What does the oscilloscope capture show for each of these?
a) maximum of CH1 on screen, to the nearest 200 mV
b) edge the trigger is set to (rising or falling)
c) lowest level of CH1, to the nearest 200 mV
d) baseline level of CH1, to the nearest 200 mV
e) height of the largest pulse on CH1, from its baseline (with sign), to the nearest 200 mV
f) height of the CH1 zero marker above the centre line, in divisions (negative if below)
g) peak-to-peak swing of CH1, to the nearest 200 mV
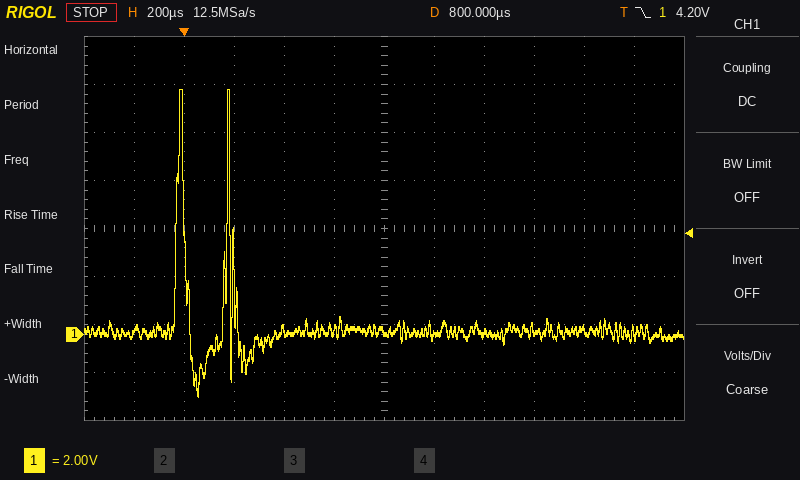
10.2 V
falling
-2.6 V
0.0 V
+10.2 V
-2.2 div
12.8 V
